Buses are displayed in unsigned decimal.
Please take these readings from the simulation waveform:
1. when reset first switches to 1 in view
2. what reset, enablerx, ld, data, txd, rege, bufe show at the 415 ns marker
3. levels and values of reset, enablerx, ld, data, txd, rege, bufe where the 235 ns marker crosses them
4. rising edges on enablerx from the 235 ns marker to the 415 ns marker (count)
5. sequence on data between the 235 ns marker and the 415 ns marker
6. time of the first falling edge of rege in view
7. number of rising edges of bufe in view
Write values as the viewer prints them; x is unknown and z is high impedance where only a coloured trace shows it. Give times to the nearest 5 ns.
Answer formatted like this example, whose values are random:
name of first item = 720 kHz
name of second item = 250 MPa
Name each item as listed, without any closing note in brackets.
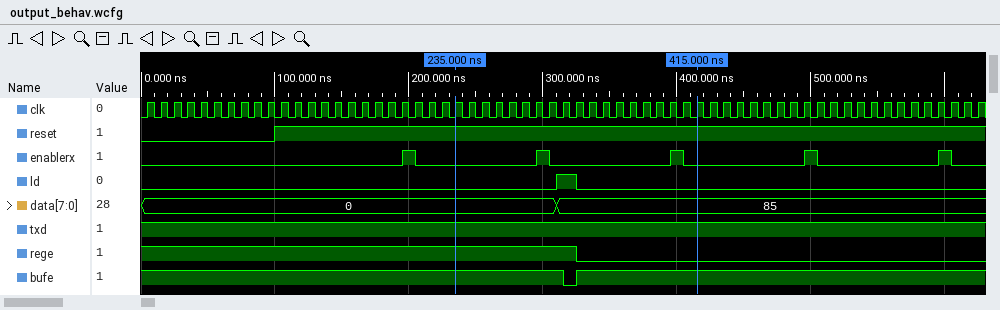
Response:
when reset first switches to 1 in view = 100 ns
what reset, enablerx, ld, data, txd, rege, bufe show at the 415 ns marker = reset=1, enablerx=0, ld=0, data=85, txd=1, rege=0, bufe=1
levels and values of reset, enablerx, ld, data, txd, rege, bufe where the 235 ns marker crosses them = reset=1, enablerx=0, ld=0, data=0, txd=1, rege=1, bufe=1
rising edges on enablerx from the 235 ns marker to the 415 ns marker = 2
sequence on data between the 235 ns marker and the 415 ns marker = 0, 85
time of the first falling edge of rege in view = 325 ns
number of rising edges of bufe in view = 1
